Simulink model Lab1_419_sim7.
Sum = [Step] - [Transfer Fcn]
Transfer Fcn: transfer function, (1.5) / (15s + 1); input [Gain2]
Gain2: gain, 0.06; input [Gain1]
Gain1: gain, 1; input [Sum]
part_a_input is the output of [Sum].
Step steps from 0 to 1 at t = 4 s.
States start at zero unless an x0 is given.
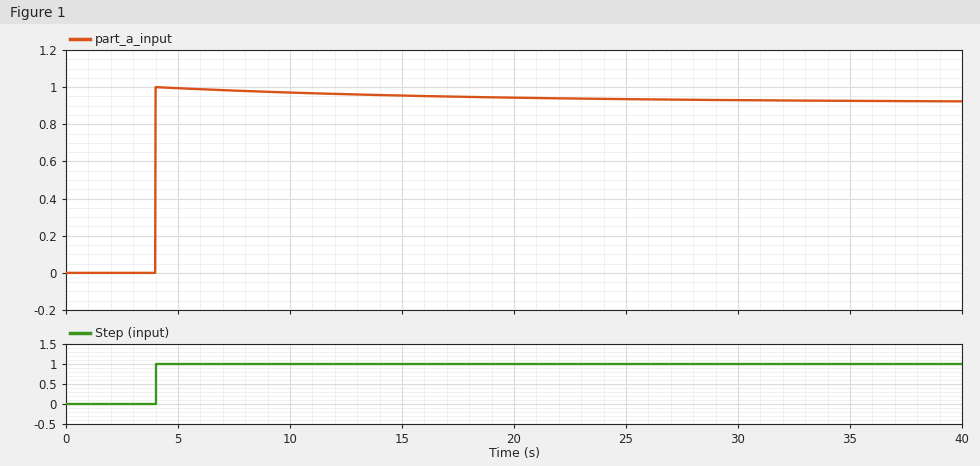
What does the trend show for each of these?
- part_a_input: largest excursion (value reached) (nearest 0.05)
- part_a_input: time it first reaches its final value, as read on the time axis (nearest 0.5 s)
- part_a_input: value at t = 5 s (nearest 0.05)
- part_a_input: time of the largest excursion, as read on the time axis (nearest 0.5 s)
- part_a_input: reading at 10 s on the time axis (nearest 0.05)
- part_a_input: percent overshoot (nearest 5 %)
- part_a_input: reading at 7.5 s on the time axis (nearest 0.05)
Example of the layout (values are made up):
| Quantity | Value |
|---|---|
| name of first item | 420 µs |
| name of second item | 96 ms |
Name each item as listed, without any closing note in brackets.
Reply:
| Quantity | Value |
|---|---|
| part_a_input: largest excursion (value reached) | 1.00 |
| part_a_input: time it first reaches its final value, as read on the time axis | 4.0 s |
| part_a_input: value at t = 5 s | 1.00 |
| part_a_input: time of the largest excursion, as read on the time axis | 4.0 s |
| part_a_input: reading at 10 s on the time axis | 0.95 |
| part_a_input: percent overshoot | 10 % |
| part_a_input: reading at 7.5 s on the time axis | 1.00 |
